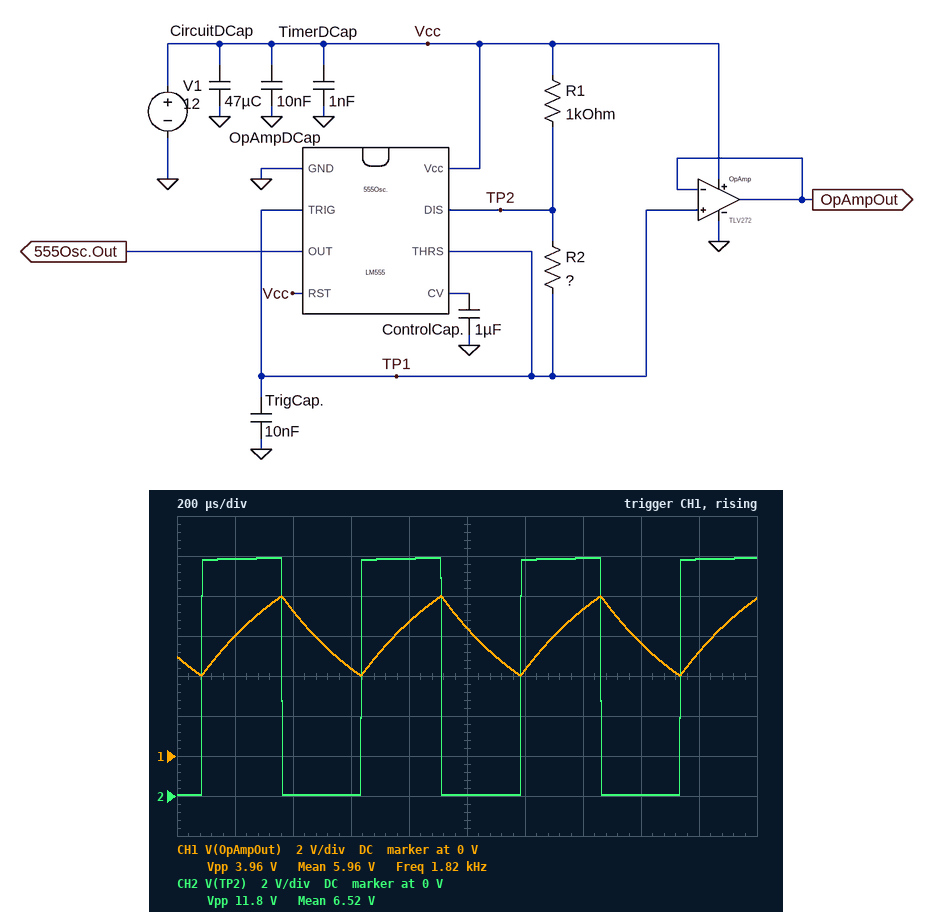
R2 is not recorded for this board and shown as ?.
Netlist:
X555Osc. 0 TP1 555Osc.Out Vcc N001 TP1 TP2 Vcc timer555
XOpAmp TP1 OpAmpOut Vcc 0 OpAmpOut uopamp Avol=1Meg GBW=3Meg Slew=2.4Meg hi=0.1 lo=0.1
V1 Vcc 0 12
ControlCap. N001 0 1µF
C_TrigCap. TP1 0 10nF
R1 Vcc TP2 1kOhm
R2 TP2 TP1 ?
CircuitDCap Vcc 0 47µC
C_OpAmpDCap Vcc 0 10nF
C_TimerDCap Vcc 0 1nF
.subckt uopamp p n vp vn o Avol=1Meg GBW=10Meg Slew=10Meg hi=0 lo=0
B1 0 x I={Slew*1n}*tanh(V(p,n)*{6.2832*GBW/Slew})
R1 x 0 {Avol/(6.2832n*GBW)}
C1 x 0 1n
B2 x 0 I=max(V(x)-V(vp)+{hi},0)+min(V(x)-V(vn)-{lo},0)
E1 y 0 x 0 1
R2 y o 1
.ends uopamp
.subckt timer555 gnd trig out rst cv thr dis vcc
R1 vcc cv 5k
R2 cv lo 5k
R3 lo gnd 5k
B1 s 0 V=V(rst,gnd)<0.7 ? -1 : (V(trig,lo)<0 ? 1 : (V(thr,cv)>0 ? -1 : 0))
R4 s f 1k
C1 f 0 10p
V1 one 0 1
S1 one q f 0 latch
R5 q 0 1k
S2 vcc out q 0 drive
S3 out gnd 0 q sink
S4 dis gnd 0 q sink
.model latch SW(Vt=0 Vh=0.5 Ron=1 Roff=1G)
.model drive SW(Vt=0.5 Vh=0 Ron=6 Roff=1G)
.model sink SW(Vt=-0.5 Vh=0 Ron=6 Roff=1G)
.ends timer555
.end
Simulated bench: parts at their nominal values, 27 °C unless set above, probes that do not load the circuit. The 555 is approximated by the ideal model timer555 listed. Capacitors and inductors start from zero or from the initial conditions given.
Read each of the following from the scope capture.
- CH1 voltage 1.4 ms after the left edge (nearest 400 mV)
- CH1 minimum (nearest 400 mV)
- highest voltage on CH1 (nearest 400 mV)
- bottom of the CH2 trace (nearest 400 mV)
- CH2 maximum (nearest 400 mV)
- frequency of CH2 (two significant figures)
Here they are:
7.2 V
4.0 V
8.0 V
0 V
12.0 V
1.8 kHz
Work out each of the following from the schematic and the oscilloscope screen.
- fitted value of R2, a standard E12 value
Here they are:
39 kΩ
